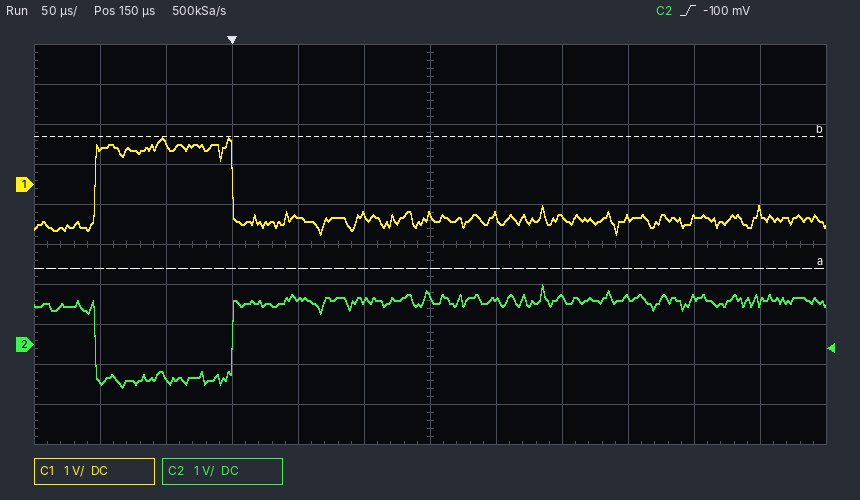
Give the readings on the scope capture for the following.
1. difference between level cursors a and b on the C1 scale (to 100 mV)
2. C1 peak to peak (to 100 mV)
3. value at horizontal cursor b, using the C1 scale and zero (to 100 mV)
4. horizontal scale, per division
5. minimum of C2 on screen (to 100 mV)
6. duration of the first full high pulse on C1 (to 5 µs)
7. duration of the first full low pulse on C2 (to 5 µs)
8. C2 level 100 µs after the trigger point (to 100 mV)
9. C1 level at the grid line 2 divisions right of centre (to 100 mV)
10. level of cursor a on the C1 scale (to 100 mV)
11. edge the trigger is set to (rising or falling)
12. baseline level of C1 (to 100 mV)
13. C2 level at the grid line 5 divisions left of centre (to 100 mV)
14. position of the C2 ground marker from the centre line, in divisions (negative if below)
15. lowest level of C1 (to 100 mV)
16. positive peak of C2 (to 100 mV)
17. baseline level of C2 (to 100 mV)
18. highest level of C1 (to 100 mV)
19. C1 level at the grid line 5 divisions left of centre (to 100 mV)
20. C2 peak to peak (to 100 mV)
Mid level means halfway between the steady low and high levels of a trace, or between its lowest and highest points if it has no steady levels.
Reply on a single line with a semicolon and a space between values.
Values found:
3.3 V; 2.4 V; 1.2 V; 50 µs; -1.1 V; 105 µs; 105 µs; 1.1 V; -800 mV; -2.1 V; rising; -900 mV; -900 mV; -2.5 div; -1.2 V; 1.5 V; 1.1 V; 1.2 V; 900 mV; 2.6 V
